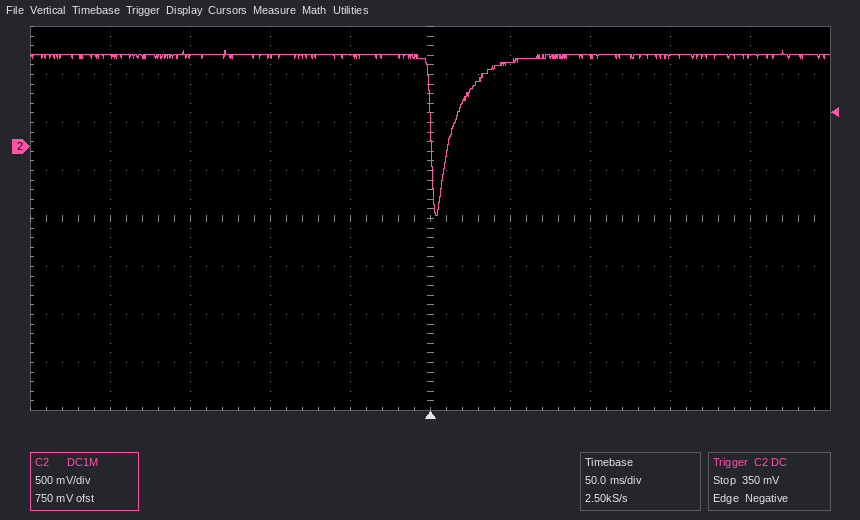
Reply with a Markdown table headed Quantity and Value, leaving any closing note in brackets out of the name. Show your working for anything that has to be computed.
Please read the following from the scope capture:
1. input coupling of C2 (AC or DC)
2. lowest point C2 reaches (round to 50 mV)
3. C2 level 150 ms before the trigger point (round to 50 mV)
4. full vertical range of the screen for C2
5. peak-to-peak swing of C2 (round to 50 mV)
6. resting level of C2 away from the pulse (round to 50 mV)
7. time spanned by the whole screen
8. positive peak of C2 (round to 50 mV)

| Quantity | Value |
|---|---|
| input coupling of C2 | DC |
| lowest point C2 reaches | -700 mV |
| C2 level 150 ms before the trigger point | 950 mV |
| full vertical range of the screen for C2 | 4 V |
| peak-to-peak swing of C2 | 1.00 V − (-700 mV) = 1.70 V |
| resting level of C2 away from the pulse | 950 mV |
| time spanned by the whole screen | 500 ms |
| positive peak of C2 | 1.00 V |
